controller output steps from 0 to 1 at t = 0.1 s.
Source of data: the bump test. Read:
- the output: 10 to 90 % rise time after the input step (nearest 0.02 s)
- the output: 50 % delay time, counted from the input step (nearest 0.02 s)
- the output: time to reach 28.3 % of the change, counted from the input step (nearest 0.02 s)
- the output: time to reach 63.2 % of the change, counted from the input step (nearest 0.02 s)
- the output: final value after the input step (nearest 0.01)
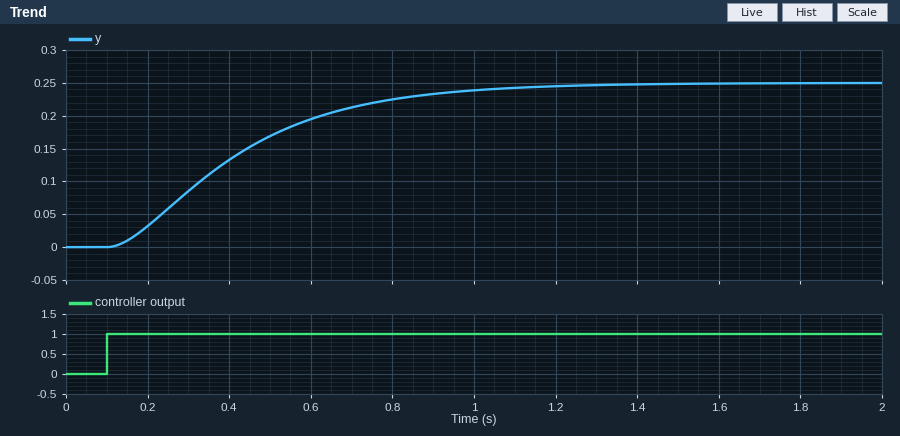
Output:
0.62 s
0.28 s
0.18 s
0.36 s
0.25
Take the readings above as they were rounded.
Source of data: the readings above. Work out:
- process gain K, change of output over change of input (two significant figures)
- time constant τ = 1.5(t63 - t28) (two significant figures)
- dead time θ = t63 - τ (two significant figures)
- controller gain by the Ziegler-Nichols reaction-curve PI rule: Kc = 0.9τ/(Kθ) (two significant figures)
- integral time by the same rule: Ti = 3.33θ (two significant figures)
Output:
0.25
0.27 s
0.090 s
11
0.30 s
